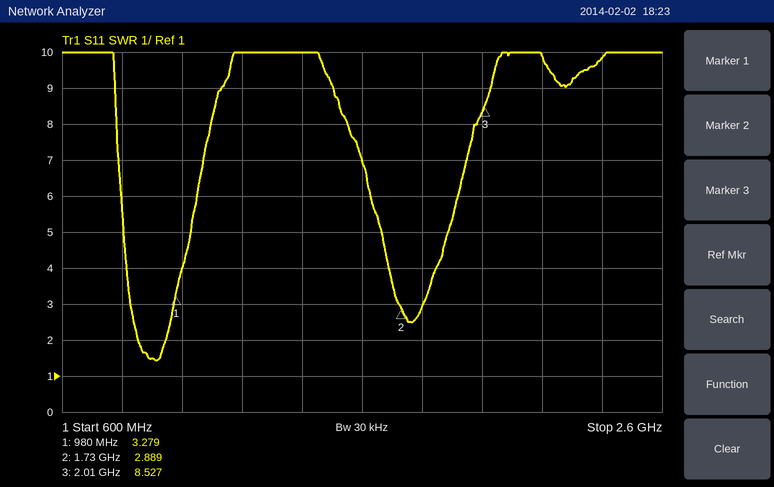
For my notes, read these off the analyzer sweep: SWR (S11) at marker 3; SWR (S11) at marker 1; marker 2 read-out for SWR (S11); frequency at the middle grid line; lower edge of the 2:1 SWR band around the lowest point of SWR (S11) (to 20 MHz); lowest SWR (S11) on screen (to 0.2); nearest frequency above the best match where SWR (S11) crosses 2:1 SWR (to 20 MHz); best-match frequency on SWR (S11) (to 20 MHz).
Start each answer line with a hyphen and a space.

- 8.527
- 3.279
- 2.889
- 1.6 GHz
- 860 MHz
- 1.4
- 940 MHz
- 920 MHz
